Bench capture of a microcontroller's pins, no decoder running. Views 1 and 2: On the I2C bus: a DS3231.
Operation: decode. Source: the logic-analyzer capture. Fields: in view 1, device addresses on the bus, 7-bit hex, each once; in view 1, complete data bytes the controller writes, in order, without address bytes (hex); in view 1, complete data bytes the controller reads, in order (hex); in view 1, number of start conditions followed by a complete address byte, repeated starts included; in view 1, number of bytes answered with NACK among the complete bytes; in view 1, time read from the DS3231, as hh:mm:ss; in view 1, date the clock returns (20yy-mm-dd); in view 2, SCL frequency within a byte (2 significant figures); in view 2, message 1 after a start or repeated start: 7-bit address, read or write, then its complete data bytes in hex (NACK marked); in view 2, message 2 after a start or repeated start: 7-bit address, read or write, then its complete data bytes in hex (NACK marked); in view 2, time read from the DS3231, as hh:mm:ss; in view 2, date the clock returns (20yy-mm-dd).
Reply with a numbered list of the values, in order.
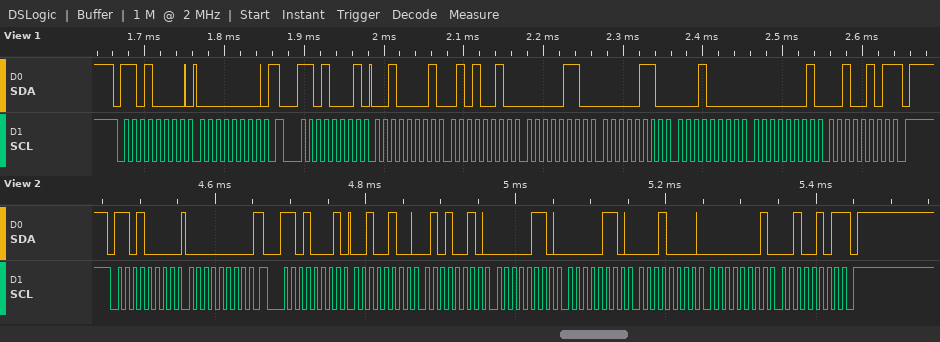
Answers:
1. 0x68
2. 00
3. 21 52 06 06 10 01 25
4. 2
5. 1
6. 06:52:21
7. 2025-01-10
8. 100 kHz
9. 0x68 write: 00
10. 0x68 read: 24 52 06 06 10 01 25 NACK
11. 06:52:24
12. 2025-01-10
